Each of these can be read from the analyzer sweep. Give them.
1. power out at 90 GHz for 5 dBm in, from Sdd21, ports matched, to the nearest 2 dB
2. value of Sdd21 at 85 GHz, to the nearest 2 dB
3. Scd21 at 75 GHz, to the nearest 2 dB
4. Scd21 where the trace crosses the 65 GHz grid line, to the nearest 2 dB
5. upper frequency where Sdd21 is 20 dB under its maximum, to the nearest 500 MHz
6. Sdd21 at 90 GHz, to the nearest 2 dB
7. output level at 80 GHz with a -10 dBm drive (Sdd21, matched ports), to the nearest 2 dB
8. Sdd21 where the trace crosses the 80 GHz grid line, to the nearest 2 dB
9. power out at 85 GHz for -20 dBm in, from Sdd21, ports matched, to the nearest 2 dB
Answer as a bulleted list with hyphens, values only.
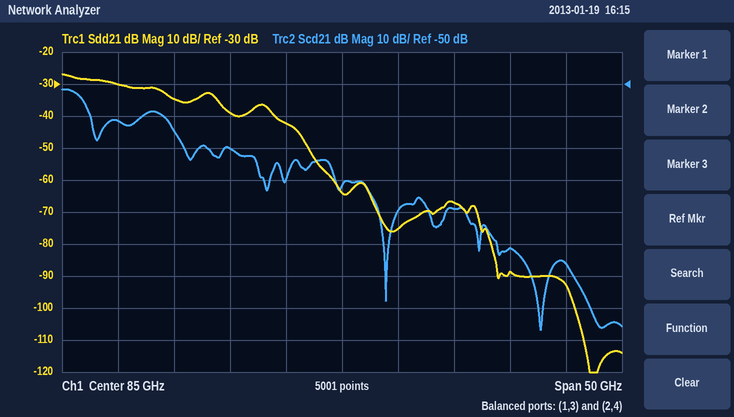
- -70 dBm
- -64 dB
- -70 dB
- -62 dB
- 81.5 GHz
- -76 dB
- -52 dBm
- -42 dB
- -84 dBm
